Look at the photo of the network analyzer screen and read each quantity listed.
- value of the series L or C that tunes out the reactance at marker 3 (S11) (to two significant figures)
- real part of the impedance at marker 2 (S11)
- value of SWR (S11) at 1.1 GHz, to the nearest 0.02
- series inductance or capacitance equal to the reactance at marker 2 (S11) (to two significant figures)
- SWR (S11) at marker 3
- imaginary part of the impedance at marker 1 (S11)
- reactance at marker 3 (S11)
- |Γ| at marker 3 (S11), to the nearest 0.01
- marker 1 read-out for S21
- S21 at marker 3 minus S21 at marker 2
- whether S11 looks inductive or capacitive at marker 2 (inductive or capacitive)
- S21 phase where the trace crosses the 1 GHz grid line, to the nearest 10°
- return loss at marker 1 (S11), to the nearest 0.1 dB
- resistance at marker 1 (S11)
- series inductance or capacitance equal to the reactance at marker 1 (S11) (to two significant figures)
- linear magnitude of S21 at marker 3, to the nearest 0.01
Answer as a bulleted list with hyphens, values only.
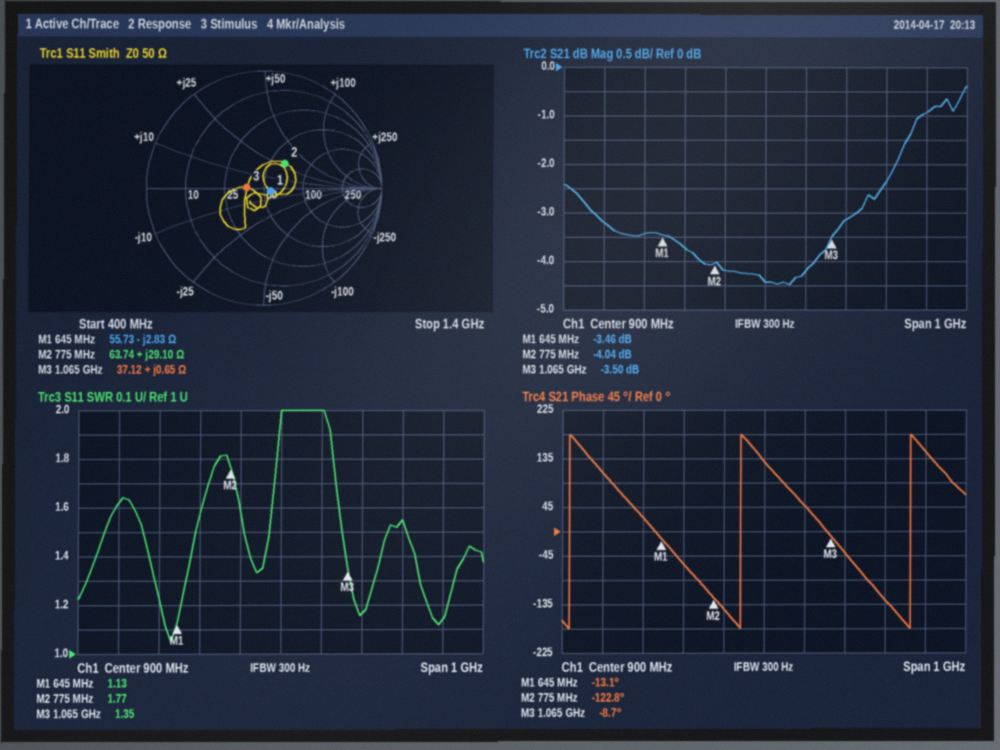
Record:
- 230 pF
- 63.74 Ω
- 1.16
- 6.0 nH
- 1.35
- -2.83 Ω
- +0.65 Ω
- 0.15
- -3.46 dB
- 0.54 dB
- inductive
- 50°
- 24.4 dB
- 55.73 Ω
- 87 pF
- 0.67
